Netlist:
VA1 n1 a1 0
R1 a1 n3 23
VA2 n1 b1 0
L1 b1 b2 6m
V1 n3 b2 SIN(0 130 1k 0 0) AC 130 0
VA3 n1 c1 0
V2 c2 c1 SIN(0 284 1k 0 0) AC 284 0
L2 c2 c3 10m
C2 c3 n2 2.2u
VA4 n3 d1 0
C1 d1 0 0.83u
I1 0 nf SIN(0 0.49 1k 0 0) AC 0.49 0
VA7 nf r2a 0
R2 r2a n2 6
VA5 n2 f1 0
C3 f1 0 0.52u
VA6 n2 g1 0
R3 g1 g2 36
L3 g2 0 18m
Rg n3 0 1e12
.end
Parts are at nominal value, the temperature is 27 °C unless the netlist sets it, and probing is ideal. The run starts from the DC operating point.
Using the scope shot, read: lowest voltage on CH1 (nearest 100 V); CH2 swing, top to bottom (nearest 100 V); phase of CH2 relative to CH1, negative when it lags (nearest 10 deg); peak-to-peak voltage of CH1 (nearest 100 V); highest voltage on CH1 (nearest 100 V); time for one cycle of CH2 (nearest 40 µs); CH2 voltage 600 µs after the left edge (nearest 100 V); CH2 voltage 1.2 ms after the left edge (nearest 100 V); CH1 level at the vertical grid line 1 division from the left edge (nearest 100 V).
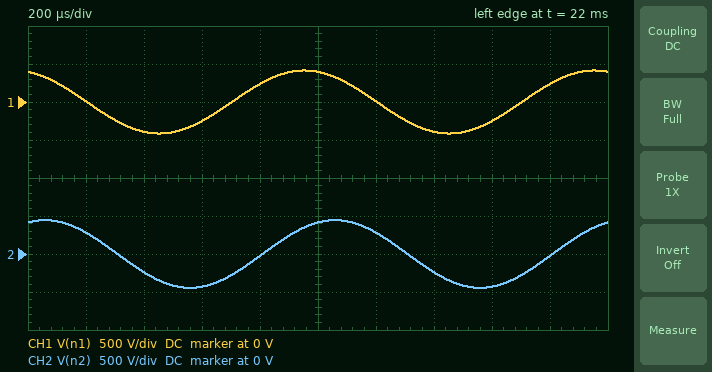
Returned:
-400 V
900 V
-40 deg
800 V
400 V
1.00 ms
-400 V
300 V
0 V
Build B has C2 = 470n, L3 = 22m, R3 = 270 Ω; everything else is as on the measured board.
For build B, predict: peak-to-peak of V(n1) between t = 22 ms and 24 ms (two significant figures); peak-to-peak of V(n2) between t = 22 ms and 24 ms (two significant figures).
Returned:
170 V
270 V
